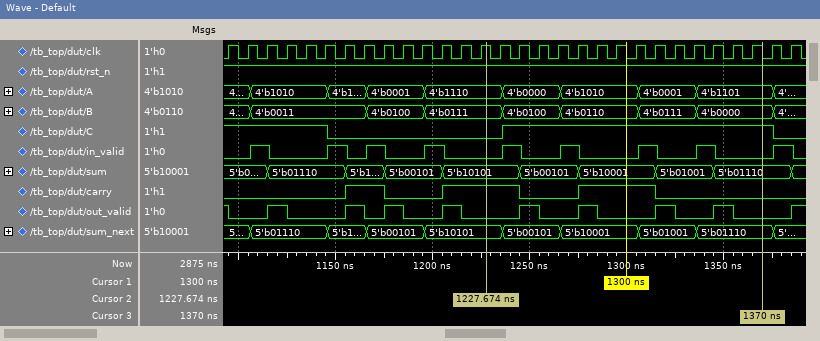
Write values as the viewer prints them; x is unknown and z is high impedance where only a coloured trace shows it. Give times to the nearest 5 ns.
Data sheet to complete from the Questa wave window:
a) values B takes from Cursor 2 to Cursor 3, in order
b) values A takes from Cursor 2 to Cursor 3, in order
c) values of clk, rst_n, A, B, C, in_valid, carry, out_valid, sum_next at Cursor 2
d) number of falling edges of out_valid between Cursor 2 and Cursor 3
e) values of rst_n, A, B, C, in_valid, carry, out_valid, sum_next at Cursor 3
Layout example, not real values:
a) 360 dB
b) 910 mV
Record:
a) 4'b0111, 4'b0100, 4'b0110, 4'b0111, 4'b0000
b) 4'b1110, 4'b0000, 4'b1010, 4'b0001, 4'b1101
c) clk=1, rst_n=1, A=4'b1110, B=4'b0111, C=0, in_valid=0, carry=1, out_valid=0, sum_next=5'b10101
d) 4
e) rst_n=1, A=4'b1101, B=4'b0000, C=1, in_valid=0, carry=0, out_valid=0, sum_next=5'b01110
